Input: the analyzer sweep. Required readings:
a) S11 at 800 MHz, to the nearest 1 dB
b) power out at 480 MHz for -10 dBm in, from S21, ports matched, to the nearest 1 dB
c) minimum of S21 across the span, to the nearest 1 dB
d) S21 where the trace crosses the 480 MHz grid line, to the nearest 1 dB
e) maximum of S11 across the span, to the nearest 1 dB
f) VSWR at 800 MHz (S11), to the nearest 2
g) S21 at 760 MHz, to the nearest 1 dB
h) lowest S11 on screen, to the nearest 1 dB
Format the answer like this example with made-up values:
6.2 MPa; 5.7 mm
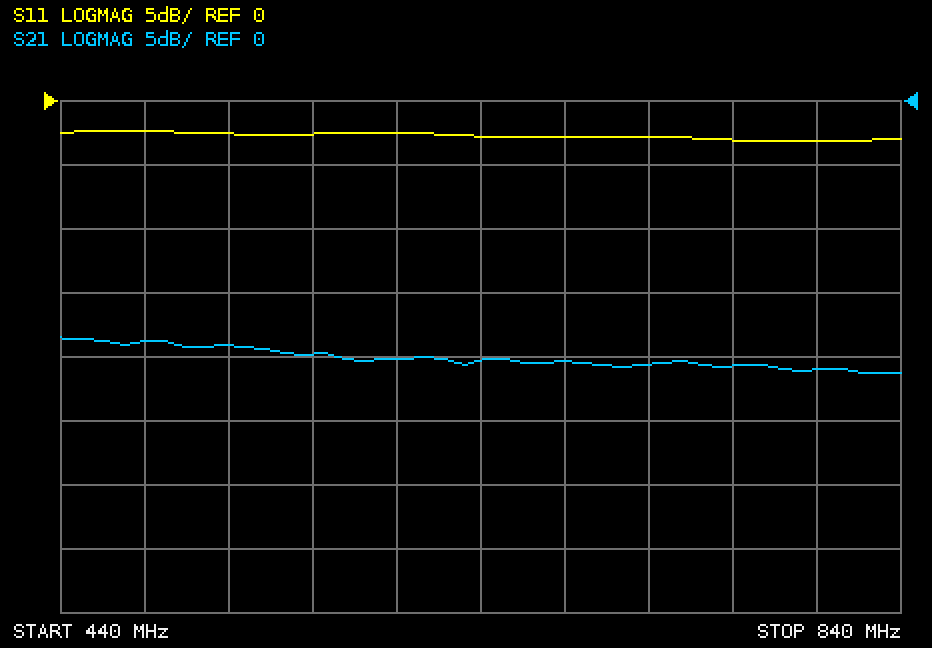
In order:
-3 dB; -29 dBm; -21 dB; -19 dB; -2 dB; 6; -21 dB; -3 dB
